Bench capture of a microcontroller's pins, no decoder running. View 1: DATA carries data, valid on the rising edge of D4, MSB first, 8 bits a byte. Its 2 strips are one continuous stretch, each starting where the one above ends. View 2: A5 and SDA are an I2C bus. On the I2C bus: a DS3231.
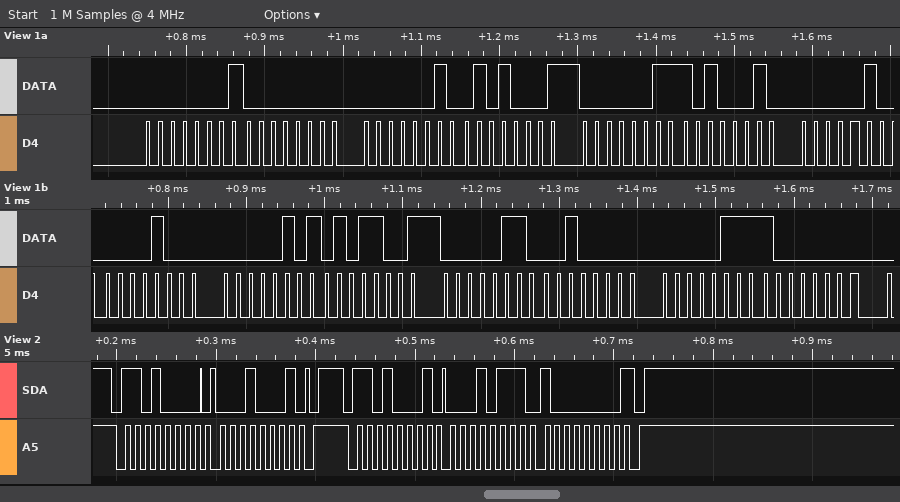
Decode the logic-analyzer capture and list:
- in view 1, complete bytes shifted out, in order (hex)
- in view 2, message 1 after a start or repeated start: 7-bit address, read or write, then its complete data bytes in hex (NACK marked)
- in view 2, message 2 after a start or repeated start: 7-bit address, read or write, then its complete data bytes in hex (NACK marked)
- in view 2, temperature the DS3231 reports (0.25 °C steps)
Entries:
0x01 0x00 0x02 0x51 0x03 0xA2 0x04 0x08 0x05 0x59 0x06 0x20 0x07 0x80
0x68 write: 11
0x68 read: 17 80 NACK
23.50 °C
